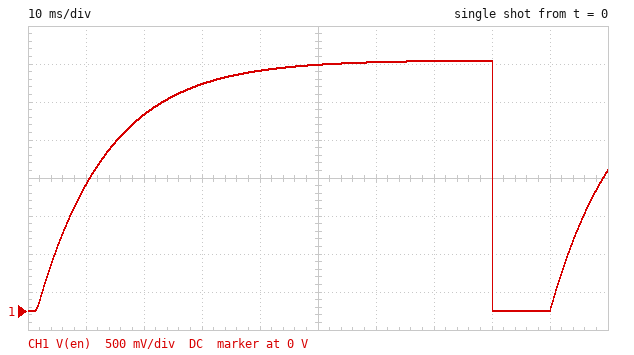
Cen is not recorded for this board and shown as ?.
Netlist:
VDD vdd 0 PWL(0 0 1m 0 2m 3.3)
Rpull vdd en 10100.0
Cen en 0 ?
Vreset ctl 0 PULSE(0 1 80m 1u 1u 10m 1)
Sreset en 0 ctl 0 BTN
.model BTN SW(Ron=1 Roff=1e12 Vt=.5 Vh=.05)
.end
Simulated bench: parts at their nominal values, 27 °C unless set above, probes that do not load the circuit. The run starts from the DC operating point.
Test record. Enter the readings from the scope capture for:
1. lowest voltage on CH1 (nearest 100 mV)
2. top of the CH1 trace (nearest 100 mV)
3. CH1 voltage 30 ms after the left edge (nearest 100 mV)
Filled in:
0 V
3.3 V
3.0 V
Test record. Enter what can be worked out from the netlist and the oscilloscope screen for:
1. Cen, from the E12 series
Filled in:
1.2 µF
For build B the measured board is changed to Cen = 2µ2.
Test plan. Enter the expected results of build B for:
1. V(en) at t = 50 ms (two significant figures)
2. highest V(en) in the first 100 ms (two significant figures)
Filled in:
2.9 V
3.2 V
